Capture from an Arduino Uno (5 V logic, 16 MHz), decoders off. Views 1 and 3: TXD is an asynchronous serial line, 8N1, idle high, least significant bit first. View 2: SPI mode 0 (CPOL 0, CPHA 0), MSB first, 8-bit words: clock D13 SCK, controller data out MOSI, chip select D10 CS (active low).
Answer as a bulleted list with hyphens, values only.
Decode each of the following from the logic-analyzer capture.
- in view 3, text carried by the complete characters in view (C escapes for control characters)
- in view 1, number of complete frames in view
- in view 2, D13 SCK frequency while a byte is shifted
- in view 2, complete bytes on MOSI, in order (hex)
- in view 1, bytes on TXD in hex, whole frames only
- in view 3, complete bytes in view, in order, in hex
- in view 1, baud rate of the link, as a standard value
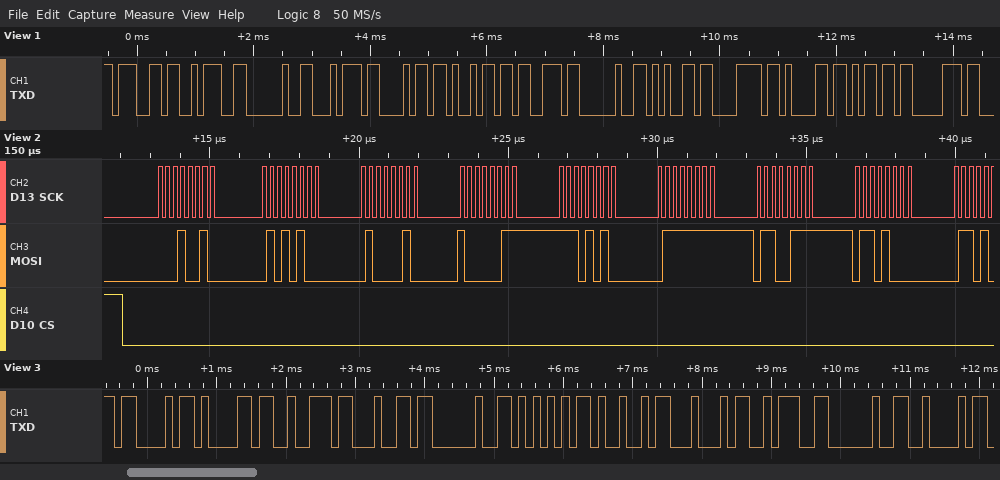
- "Card UID: B"
- 13
- 4 MHz
- 0x12 0x54 0x42 0x83 0xEA 0x7F 0x67 0x68
- 67 3A 20 74 68 69 73 20 65 78 61 6D 70
- 43 61 72 64 20 55 49 44 3A 20 42
- 9600 baud
